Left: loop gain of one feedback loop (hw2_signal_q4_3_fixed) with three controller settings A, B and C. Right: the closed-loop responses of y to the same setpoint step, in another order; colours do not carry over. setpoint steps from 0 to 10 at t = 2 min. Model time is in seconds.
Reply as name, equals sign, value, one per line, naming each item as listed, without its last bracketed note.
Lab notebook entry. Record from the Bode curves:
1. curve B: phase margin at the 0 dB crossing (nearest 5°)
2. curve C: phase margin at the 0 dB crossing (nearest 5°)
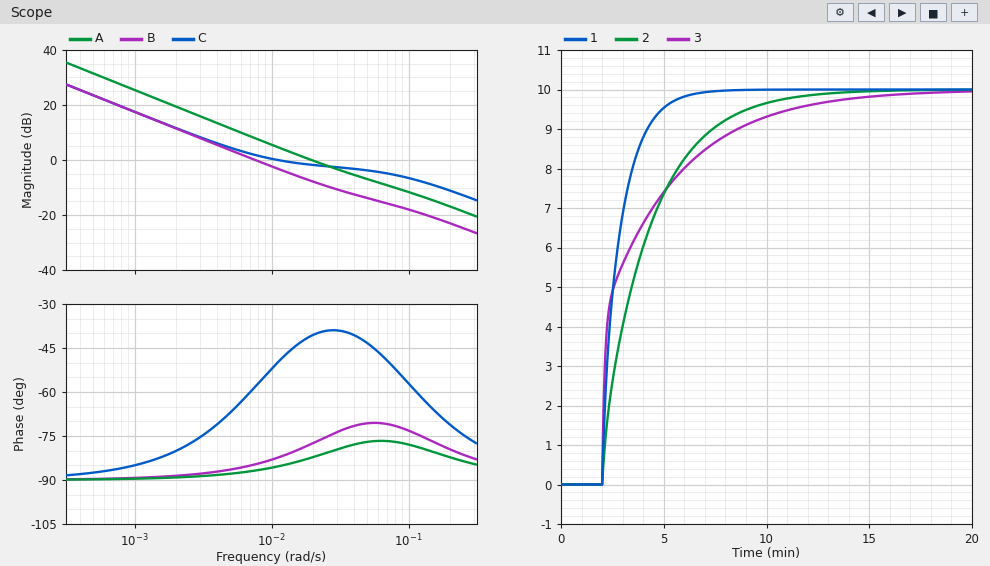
curve B: phase margin at the 0 dB crossing = 95°
curve C: phase margin at the 0 dB crossing = 130°
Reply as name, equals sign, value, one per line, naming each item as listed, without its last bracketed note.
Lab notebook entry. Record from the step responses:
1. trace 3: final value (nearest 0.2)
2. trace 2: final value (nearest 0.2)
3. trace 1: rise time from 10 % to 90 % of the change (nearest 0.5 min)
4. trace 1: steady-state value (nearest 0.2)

trace 3: final value = 10.0
trace 2: final value = 10.0
trace 1: rise time from 10 % to 90 % of the change = 2.0 min
trace 1: steady-state value = 10.0
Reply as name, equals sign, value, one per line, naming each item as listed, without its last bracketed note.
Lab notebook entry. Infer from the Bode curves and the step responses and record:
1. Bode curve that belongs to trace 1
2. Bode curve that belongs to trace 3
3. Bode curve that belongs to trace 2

Bode curve that belongs to trace 1 = A
Bode curve that belongs to trace 3 = C
Bode curve that belongs to trace 2 = B
